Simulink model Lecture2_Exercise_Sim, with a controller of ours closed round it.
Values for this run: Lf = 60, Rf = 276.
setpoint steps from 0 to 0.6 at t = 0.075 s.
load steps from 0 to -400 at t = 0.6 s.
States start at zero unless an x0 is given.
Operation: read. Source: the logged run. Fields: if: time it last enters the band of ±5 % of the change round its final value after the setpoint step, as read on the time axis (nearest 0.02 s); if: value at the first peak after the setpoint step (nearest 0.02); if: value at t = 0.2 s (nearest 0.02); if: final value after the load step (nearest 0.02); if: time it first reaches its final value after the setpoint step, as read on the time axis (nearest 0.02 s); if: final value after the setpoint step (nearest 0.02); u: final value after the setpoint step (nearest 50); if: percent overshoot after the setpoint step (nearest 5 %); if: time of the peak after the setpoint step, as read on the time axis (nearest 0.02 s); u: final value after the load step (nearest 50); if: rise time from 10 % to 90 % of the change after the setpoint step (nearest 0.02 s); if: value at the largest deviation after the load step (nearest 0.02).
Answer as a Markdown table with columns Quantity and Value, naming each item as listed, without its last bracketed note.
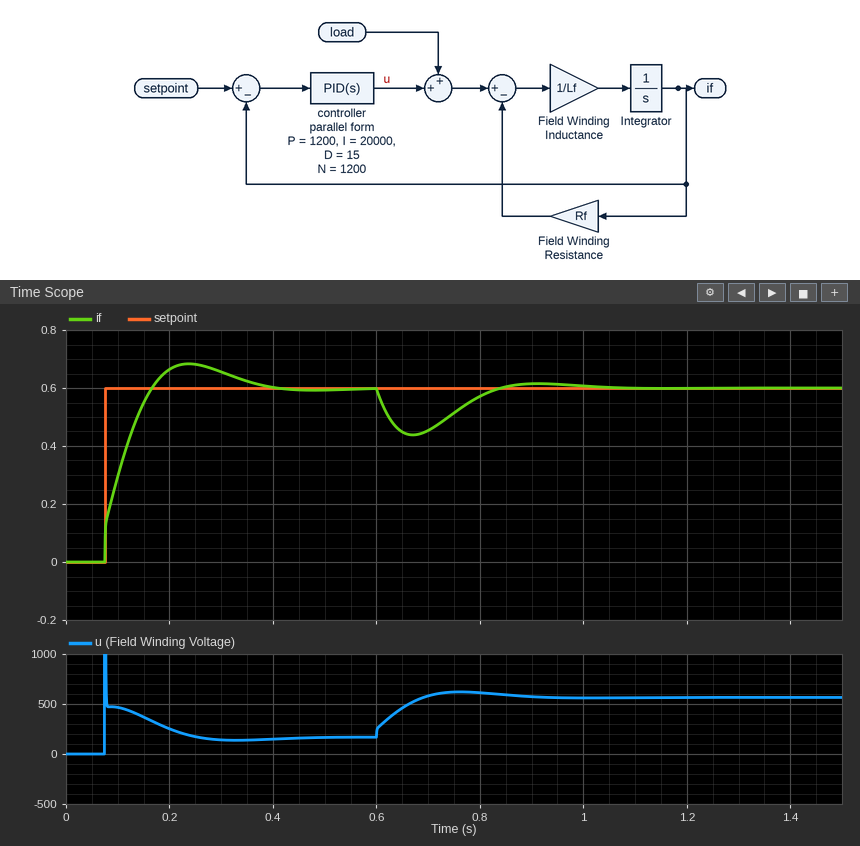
| Quantity | Value |
|---|---|
| if: time it last enters the band of ±5 % of the change round its final value after the setpoint step, as read on the time axis | 0.34 s |
| if: value at the first peak after the setpoint step | 0.68 |
| if: value at t = 0.2 s | 0.66 |
| if: final value after the load step | 0.60 |
| if: time it first reaches its final value after the setpoint step, as read on the time axis | 0.16 s |
| if: final value after the setpoint step | 0.60 |
| u: final value after the setpoint step | 150 |
| if: percent overshoot after the setpoint step | 15 % |
| if: time of the peak after the setpoint step, as read on the time axis | 0.24 s |
| u: final value after the load step | 550 |
| if: rise time from 10 % to 90 % of the change after the setpoint step | 0.08 s |
| if: value at the largest deviation after the load step | 0.44 |
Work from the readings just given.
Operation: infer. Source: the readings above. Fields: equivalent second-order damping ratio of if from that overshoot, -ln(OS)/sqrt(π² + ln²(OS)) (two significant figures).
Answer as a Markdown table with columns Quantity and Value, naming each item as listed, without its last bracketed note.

| Quantity | Value |
|---|---|
| equivalent second-order damping ratio of if from that overshoot, -ln(OS)/sqrt(π² + ln²(OS)) | 0.52 |
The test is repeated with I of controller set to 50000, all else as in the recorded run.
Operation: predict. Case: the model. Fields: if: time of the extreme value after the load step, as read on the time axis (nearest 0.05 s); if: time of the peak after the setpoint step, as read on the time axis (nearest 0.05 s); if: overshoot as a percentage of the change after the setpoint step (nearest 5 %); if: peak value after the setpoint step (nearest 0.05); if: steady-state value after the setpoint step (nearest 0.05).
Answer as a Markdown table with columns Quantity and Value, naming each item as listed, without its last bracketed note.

| Quantity | Value |
|---|---|
| if: time of the extreme value after the load step, as read on the time axis | 0.65 s |
| if: time of the peak after the setpoint step, as read on the time axis | 0.20 s |
| if: overshoot as a percentage of the change after the setpoint step | 25 % |
| if: peak value after the setpoint step | 0.75 |
| if: steady-state value after the setpoint step | 0.60 |
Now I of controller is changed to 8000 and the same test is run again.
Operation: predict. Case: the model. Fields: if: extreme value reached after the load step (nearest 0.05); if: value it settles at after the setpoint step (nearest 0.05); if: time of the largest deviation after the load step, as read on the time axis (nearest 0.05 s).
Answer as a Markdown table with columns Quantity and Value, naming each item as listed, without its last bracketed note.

| Quantity | Value |
|---|---|
| if: extreme value reached after the load step | 0.40 |
| if: value it settles at after the setpoint step | 0.60 |
| if: time of the largest deviation after the load step, as read on the time axis | 0.70 s |
